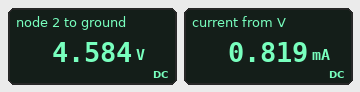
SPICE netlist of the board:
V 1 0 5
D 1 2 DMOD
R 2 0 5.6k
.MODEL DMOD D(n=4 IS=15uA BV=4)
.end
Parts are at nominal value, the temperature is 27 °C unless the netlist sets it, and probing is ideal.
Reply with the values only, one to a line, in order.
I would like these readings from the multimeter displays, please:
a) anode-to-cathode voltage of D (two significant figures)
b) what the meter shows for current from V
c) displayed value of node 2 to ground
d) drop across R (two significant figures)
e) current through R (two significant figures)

420 mV
0.819 mA
4.584 V
4.6 V
820 µA
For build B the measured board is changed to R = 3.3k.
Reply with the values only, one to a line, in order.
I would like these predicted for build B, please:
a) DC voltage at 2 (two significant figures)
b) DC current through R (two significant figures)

4.5 V
1.4 mA
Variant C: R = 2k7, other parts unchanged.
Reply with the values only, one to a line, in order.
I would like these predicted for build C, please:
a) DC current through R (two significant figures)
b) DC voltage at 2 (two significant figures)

1.7 mA
4.5 V
